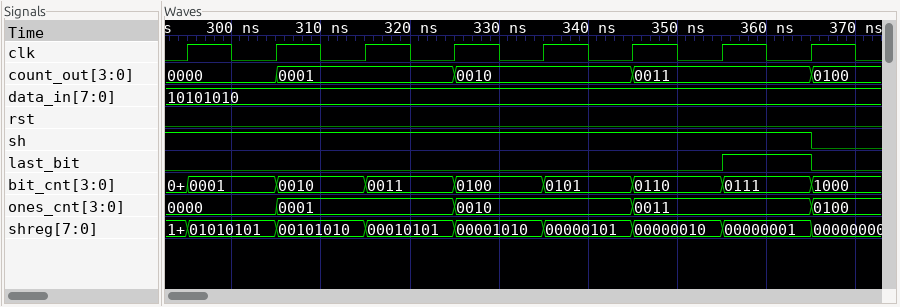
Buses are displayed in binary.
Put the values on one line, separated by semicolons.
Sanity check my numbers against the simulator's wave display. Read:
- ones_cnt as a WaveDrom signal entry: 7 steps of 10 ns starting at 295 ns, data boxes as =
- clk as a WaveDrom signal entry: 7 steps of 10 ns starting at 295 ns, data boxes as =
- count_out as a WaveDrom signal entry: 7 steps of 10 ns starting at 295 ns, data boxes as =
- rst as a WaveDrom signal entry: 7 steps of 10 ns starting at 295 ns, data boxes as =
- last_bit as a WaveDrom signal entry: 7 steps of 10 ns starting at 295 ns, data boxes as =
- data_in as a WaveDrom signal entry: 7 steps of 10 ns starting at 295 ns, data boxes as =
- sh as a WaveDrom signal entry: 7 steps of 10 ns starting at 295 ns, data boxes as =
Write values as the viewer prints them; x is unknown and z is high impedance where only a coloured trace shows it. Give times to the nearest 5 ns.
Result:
{name: 'ones_cnt', wave: '==.=.=.', data: '0000 0001 0010 0011'}; {name: 'clk', wave: 'p......'}; {name: 'count_out', wave: '==.=.=.', data: '0000 0001 0010 0011'}; {name: 'rst', wave: '0......'}; {name: 'last_bit', wave: '0.....1'}; {name: 'data_in', wave: '=......', data: '10101010'}; {name: 'sh', wave: '1......'}
